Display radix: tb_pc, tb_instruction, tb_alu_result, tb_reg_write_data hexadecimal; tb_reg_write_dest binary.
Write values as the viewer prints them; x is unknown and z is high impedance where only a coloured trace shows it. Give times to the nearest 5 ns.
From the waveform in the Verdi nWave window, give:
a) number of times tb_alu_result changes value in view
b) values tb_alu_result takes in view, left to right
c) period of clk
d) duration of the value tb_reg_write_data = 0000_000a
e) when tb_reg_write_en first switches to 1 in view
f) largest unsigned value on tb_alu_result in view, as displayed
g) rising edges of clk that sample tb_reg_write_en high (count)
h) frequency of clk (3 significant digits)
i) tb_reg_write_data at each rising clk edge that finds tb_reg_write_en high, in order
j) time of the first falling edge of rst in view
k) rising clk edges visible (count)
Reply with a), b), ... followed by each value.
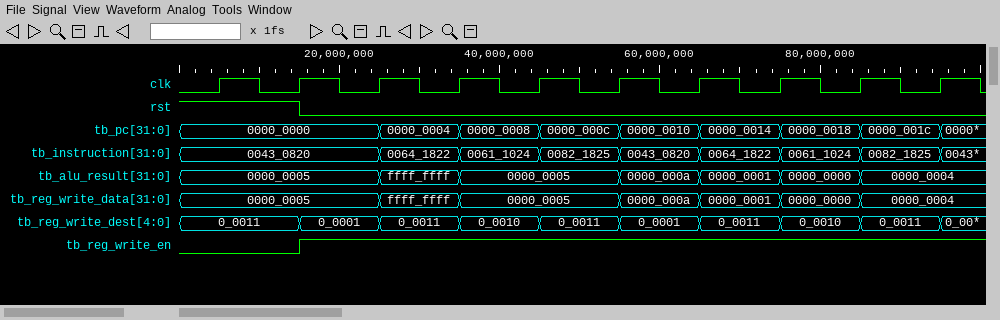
a) 6
b) 0000_0005, ffff_ffff, 0000_0005, 0000_000a, 0000_0001, 0000_0000, 0000_0004
c) 10 ns
d) 10 ns
e) 15 ns
f) ffff_ffff
g) 8
h) 100 MHz
i) 0000_0005, ffff_ffff, 0000_0005, 0000_0005, 0000_000a, 0000_0001, 0000_0000, 0000_0004
j) 15 ns
k) 10
